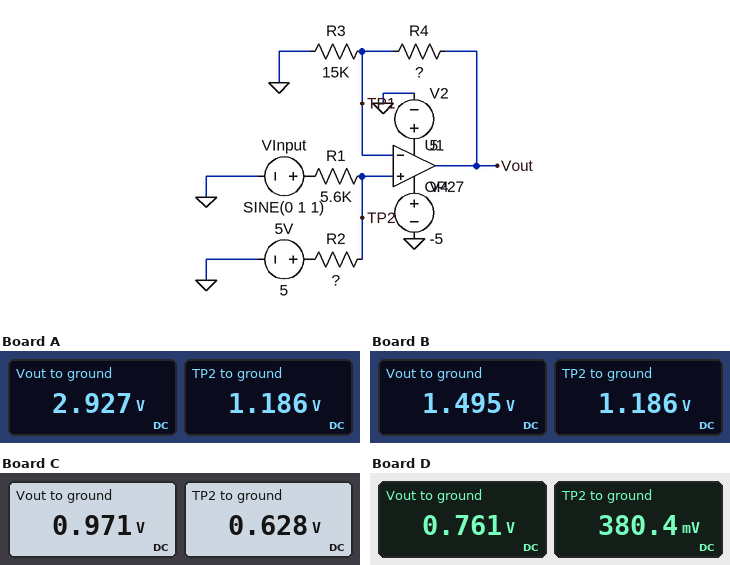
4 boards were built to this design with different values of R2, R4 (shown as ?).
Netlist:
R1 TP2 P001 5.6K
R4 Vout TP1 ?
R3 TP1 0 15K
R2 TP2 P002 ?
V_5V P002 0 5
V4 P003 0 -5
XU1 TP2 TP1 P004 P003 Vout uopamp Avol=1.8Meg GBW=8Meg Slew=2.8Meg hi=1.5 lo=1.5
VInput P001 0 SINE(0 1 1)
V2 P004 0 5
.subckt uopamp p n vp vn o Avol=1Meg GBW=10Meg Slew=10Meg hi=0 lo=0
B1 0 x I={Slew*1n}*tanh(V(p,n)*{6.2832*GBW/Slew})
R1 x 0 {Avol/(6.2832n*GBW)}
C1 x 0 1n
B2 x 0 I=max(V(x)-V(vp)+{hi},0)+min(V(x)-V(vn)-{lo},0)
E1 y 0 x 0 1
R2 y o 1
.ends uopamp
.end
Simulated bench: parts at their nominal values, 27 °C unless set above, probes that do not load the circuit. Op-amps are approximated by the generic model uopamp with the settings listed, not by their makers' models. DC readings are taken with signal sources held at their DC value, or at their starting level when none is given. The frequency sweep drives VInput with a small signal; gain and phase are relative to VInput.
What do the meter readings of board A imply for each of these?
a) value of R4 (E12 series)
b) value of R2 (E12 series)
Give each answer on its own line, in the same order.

22 kΩ
18 kΩ
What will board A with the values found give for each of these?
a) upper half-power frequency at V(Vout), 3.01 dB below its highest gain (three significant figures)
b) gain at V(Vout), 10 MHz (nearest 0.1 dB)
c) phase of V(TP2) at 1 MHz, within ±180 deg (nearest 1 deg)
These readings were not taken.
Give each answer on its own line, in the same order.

3.24 MHz
-4.7 dB
0 deg
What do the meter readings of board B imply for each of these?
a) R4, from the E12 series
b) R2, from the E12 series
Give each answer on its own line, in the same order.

3.9 kΩ
18 kΩ
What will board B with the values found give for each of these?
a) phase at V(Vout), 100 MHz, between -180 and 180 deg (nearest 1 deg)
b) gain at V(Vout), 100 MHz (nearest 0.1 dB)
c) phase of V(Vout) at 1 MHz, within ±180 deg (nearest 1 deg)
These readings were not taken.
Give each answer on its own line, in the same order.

-86 deg
-24.3 dB
-9 deg
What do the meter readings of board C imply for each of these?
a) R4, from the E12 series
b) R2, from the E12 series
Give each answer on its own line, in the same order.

8.2 kΩ
39 kΩ
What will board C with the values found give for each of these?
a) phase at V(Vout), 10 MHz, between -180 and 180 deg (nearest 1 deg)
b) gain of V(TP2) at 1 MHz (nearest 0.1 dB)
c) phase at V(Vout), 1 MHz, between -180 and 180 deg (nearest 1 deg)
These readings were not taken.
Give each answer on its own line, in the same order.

-63 deg
-1.2 dB
-11 deg
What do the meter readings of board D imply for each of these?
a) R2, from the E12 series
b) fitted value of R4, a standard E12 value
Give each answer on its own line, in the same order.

68 kΩ
15 kΩ
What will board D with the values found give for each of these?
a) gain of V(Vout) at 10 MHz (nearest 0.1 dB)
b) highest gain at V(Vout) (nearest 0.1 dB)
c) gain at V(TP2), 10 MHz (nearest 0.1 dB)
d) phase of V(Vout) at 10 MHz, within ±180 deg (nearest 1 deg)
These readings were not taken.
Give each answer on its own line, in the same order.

-3.3 dB
5.3 dB
-0.7 dB
-68 deg
